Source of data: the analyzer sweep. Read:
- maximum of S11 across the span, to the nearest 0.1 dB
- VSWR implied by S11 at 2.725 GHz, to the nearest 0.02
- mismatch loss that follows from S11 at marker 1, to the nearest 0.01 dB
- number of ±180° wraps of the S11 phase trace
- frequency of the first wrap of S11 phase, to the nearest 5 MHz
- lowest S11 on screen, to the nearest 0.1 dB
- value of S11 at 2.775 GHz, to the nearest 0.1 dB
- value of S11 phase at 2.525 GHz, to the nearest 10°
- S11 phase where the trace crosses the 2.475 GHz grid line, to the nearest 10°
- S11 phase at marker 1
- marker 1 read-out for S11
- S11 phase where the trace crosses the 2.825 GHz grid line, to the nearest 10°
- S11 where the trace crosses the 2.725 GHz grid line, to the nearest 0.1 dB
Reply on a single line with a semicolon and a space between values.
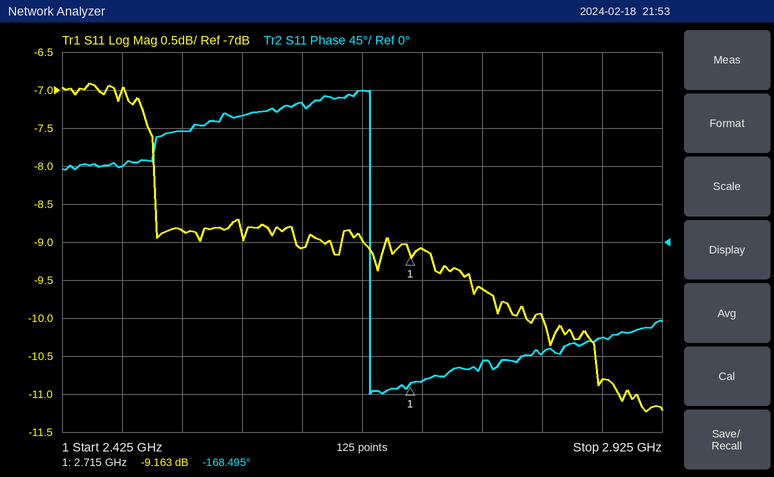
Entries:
-6.9 dB; 2.08; 0.56 dB; 1; 2.680 GHz; -11.2 dB; -9.6 dB; 130°; 90°; -168.495°; -9.163 dB; -130°; -9.1 dB
